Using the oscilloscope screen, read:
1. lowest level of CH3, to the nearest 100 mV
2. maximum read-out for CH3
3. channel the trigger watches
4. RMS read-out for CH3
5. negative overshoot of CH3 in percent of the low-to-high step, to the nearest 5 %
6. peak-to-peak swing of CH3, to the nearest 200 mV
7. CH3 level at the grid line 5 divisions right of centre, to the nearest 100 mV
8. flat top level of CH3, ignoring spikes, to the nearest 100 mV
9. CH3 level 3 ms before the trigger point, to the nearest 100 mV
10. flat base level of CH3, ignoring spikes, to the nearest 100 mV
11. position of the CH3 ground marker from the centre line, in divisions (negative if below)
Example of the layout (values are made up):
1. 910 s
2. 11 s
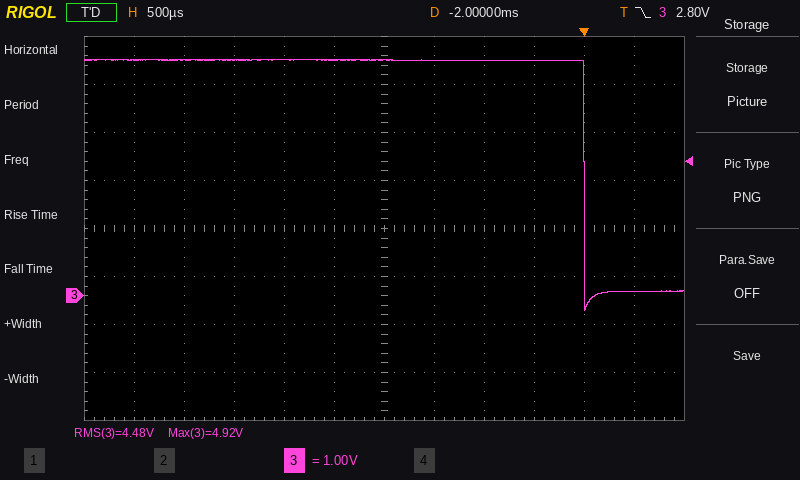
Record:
1. -300 mV
2. 4.92 V
3. CH3
4. 4.48 V
5. 10 %
6. 5.2 V
7. 100 mV
8. 4.9 V
9. 4.9 V
10. 100 mV
11. -1.4 div
